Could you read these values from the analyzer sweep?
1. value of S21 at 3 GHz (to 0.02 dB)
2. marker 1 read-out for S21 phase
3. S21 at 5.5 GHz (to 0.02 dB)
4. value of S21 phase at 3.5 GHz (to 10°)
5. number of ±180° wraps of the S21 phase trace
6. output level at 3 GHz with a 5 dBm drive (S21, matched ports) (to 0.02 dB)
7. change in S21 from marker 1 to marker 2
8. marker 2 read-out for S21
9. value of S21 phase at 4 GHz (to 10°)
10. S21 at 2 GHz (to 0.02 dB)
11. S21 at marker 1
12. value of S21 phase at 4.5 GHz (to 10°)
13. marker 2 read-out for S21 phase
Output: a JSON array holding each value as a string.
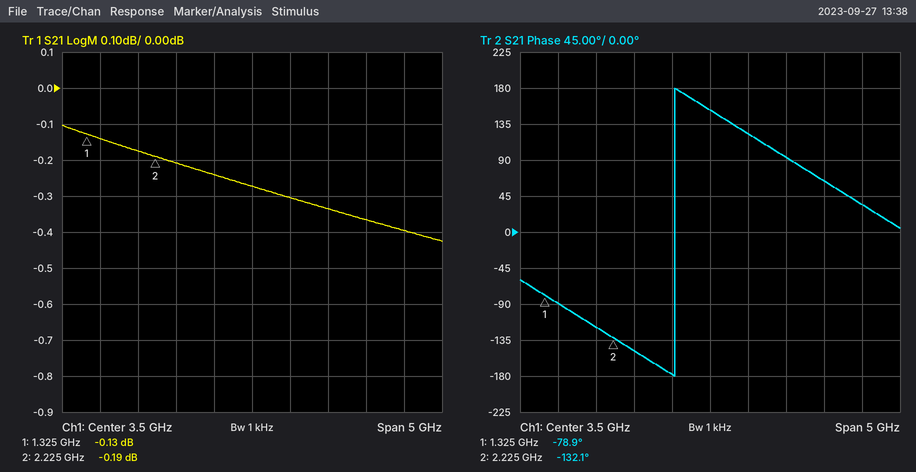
["-0.24 dB", "-78.9°", "-0.40 dB", "150°", "1", "4.76 dBm", "-0.06 dB", "-0.19 dB", "120°", "-0.18 dB", "-0.13 dB", "90°", "-132.1°"]
